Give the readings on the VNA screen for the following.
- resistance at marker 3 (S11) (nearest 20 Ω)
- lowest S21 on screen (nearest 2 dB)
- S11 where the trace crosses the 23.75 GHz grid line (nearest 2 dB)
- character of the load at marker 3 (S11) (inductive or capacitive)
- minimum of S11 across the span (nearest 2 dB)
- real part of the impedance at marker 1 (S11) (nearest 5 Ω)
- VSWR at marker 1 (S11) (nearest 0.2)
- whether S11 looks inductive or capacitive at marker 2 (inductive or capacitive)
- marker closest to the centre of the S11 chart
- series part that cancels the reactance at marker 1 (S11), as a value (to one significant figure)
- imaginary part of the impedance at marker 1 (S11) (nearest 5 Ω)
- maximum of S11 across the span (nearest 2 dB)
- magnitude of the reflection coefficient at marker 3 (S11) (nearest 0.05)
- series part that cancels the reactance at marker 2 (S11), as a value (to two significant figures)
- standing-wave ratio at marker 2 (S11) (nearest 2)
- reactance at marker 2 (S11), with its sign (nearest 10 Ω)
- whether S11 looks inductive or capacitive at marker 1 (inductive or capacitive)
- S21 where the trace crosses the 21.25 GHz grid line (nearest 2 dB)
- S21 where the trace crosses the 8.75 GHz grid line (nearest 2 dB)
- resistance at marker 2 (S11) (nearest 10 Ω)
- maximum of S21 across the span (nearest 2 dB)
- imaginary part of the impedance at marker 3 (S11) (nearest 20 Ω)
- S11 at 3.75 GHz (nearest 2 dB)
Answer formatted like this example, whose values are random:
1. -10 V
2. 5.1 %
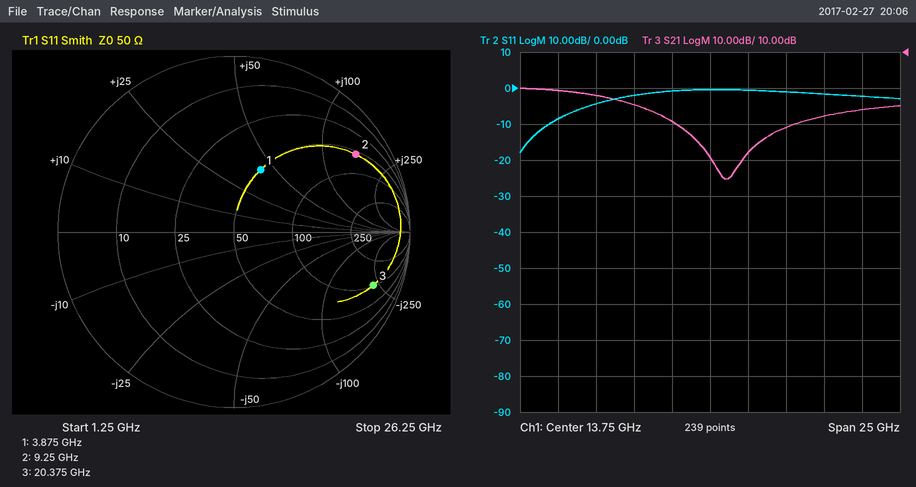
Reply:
1. 100 Ω
2. -26 dB
3. -2 dB
4. capacitive
5. -18 dB
6. 50 Ω
7. 2.2
8. inductive
9. marker 1
10. 1.0 pF
11. +40 Ω
12. 0 dB
13. 0.85
14. 110 fF
15. 10
16. +150 Ω
17. inductive
18. -8 dB
19. -4 dB
20. 60 Ω
21. 0 dB
22. -220 Ω
23. -8 dB
